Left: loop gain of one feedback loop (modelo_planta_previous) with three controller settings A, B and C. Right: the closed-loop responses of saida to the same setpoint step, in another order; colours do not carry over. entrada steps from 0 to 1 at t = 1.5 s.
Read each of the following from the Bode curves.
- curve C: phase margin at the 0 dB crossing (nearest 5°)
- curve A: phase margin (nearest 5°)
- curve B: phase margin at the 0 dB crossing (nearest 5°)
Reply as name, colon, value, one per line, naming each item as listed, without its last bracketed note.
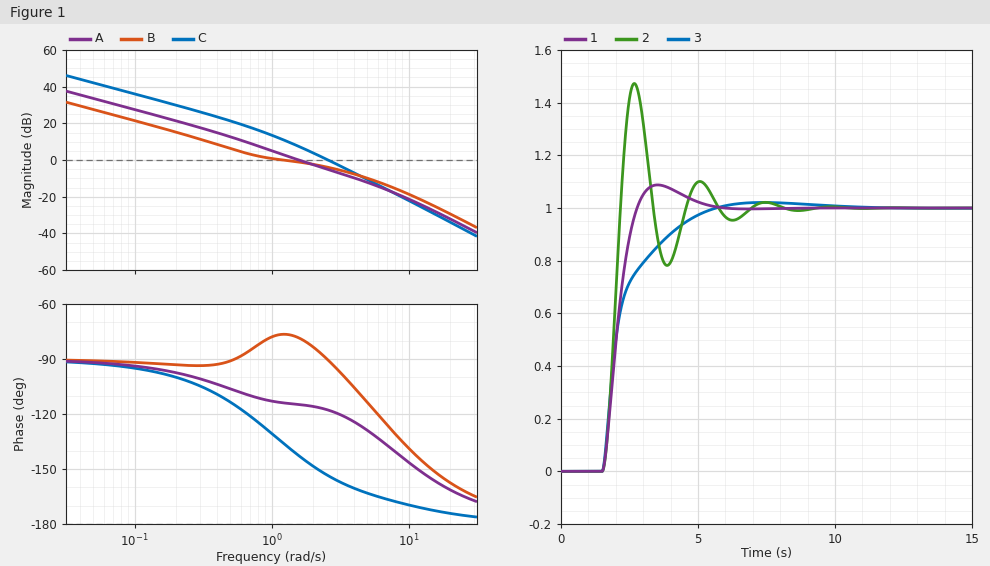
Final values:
curve C: phase margin at the 0 dB crossing: 25°
curve A: phase margin: 65°
curve B: phase margin at the 0 dB crossing: 105°
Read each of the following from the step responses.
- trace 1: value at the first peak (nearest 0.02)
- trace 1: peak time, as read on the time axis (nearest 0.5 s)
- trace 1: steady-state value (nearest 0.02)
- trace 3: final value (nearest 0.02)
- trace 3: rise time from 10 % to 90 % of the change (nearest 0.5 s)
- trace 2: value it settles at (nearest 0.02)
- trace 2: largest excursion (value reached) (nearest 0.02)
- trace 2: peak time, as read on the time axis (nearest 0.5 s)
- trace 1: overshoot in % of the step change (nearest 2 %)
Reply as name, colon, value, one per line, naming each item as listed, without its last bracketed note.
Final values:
trace 1: value at the first peak: 1.08
trace 1: peak time, as read on the time axis: 3.5 s
trace 1: steady-state value: 1.00
trace 3: final value: 1.00
trace 3: rise time from 10 % to 90 % of the change: 2.5 s
trace 2: value it settles at: 1.00
trace 2: largest excursion (value reached): 1.48
trace 2: peak time, as read on the time axis: 2.5 s
trace 1: overshoot in % of the step change: 8 %
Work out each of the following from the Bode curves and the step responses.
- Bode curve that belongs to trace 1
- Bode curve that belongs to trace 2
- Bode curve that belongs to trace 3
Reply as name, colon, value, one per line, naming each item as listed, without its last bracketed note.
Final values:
Bode curve that belongs to trace 1: A
Bode curve that belongs to trace 2: C
Bode curve that belongs to trace 3: B
